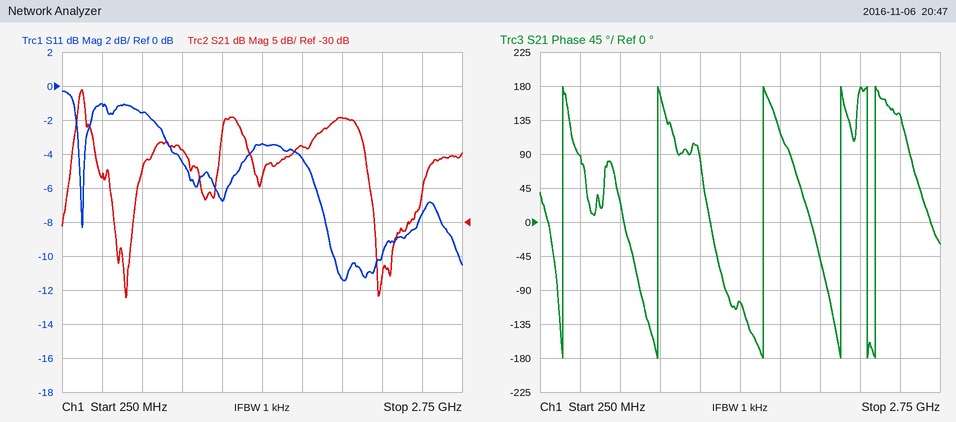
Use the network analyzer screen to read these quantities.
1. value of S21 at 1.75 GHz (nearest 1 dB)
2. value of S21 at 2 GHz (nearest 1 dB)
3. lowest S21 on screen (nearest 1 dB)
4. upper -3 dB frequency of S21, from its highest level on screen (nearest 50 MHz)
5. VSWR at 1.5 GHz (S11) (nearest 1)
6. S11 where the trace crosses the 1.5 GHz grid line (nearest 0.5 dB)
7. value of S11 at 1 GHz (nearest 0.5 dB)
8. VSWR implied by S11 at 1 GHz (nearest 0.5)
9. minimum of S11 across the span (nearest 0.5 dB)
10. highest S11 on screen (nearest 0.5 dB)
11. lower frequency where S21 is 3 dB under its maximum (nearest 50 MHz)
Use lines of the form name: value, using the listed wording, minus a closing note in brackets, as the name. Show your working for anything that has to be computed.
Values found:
value of S21 at 1.75 GHz: -19 dB
value of S21 at 2 GHz: -15 dB
lowest S21 on screen: -41 dB
upper -3 dB frequency of S21, from its highest level on screen: 400 MHz
VSWR at 1.5 GHz (S11): |Γ| = 10^(-3.5/20) = 0.6683; VSWR = (1 + 0.6683)/(1 − 0.6683) ≈ 5
S11 where the trace crosses the 1.5 GHz grid line: -3.5 dB
value of S11 at 1 GHz: -4.5 dB
VSWR implied by S11 at 1 GHz: |Γ| = 10^(-4.5/20) = 0.5957; VSWR = (1 + 0.5957)/(1 − 0.5957) ≈ 4.0
minimum of S11 across the span: -11.5 dB
highest S11 on screen: -0.5 dB
lower frequency where S21 is 3 dB under its maximum: 350 MHz
